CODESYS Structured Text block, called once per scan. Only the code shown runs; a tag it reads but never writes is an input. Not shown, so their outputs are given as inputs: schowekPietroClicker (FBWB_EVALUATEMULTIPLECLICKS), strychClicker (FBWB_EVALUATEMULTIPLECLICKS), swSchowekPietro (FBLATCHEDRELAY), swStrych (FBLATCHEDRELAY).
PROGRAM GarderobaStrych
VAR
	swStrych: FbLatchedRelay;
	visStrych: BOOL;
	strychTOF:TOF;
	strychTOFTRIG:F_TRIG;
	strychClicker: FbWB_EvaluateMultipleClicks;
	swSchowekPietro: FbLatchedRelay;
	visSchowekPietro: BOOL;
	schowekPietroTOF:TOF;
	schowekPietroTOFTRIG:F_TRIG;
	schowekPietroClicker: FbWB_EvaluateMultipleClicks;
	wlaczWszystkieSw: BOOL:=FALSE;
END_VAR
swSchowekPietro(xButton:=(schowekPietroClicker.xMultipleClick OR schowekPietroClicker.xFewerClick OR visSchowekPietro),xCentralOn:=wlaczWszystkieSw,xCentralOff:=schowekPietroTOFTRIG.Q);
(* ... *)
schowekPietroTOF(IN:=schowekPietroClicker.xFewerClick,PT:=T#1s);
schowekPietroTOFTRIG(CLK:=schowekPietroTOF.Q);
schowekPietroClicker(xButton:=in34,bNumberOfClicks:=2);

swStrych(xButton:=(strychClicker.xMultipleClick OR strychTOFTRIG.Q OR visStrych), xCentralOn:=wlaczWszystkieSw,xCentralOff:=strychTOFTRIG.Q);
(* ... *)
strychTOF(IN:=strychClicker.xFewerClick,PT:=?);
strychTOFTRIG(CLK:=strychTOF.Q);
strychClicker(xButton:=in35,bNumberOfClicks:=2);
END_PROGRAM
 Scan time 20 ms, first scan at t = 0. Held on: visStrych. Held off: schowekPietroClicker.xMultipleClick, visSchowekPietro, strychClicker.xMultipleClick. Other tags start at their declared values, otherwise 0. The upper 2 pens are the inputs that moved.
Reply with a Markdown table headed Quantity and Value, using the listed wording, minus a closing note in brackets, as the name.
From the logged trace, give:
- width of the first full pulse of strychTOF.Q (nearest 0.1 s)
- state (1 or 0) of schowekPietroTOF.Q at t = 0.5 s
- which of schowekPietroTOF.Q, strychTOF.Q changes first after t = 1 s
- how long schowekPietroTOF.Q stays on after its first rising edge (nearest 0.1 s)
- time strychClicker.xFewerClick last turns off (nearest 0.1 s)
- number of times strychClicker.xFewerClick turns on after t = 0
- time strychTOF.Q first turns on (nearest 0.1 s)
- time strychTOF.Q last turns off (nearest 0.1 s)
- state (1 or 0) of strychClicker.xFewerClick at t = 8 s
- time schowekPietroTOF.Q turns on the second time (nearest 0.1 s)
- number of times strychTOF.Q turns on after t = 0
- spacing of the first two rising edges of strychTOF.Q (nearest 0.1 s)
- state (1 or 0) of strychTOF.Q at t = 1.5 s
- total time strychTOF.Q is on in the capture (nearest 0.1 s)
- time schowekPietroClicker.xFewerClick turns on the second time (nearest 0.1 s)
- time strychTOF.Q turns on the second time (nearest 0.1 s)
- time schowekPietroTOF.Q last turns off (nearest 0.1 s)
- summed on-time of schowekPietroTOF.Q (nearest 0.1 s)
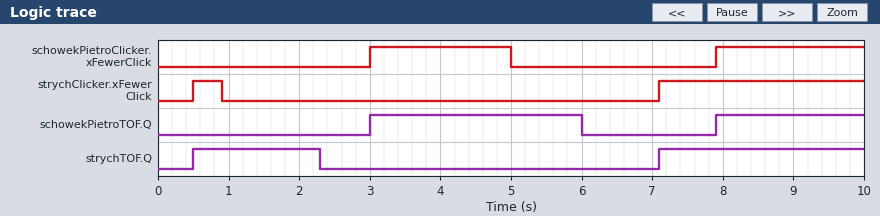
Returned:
| Quantity | Value |
|---|---|
| width of the first full pulse of strychTOF.Q | 1.8 s |
| state (1 or 0) of schowekPietroTOF.Q at t = 0.5 s | 0 |
| which of schowekPietroTOF.Q, strychTOF.Q changes first after t = 1 s | strychTOF.Q |
| how long schowekPietroTOF.Q stays on after its first rising edge | 3.0 s |
| time strychClicker.xFewerClick last turns off | 0.9 s |
| number of times strychClicker.xFewerClick turns on after t = 0 | 2 |
| time strychTOF.Q first turns on | 0.5 s |
| time strychTOF.Q last turns off | 2.3 s |
| state (1 or 0) of strychClicker.xFewerClick at t = 8 s | 1 |
| time schowekPietroTOF.Q turns on the second time | 7.9 s |
| number of times strychTOF.Q turns on after t = 0 | 2 |
| spacing of the first two rising edges of strychTOF.Q | 6.6 s |
| state (1 or 0) of strychTOF.Q at t = 1.5 s | 1 |
| total time strychTOF.Q is on in the capture | 4.7 s |
| time schowekPietroClicker.xFewerClick turns on the second time | 7.9 s |
| time strychTOF.Q turns on the second time | 7.1 s |
| time schowekPietroTOF.Q last turns off | 6.0 s |
| summed on-time of schowekPietroTOF.Q | 5.1 s |
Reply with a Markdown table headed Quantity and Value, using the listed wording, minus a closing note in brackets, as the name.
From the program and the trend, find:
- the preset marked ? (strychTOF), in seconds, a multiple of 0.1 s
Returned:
| Quantity | Value |
|---|---|
| the preset marked ? (strychTOF), in seconds, a multiple of 0.1 s | 1.4 s |
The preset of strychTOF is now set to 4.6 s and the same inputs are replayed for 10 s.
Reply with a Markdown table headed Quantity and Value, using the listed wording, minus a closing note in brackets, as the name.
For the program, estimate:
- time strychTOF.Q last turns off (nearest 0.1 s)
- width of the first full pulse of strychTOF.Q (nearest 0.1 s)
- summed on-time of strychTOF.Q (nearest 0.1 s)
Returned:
| Quantity | Value |
|---|---|
| time strychTOF.Q last turns off | 5.5 s |
| width of the first full pulse of strychTOF.Q | 5.0 s |
| summed on-time of strychTOF.Q | 7.9 s |
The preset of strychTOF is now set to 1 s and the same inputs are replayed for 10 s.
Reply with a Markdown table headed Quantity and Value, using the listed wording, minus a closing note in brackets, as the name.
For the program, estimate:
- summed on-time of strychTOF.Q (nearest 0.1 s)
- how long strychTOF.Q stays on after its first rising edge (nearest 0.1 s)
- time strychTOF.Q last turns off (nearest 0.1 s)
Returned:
| Quantity | Value |
|---|---|
| summed on-time of strychTOF.Q | 4.3 s |
| how long strychTOF.Q stays on after its first rising edge | 1.4 s |
| time strychTOF.Q last turns off | 1.9 s |
